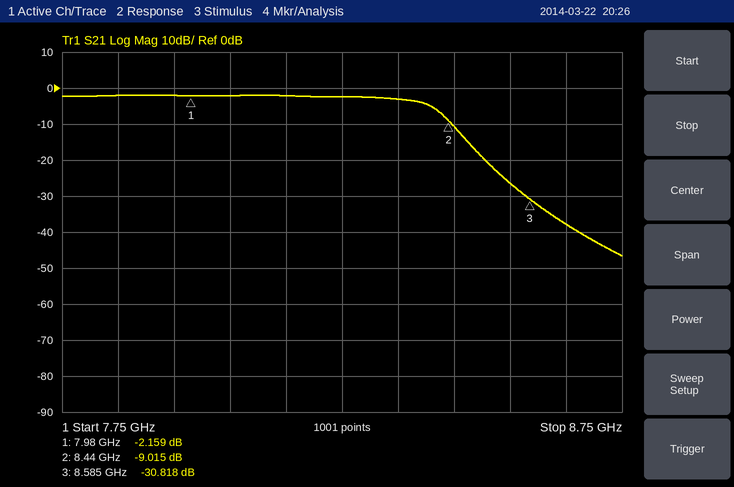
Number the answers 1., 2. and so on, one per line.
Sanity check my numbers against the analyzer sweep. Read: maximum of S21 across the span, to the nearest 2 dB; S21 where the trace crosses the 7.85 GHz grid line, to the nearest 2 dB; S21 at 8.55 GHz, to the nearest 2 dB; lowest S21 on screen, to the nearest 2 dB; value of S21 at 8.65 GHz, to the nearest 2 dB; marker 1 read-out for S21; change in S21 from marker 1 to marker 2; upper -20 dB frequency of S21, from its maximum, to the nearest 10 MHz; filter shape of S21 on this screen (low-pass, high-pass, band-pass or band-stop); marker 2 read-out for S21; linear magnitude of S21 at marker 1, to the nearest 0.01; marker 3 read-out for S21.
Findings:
1. -2 dB
2. -2 dB
3. -26 dB
4. -46 dB
5. -38 dB
6. -2.159 dB
7. -6.856 dB
8. 8.52 GHz
9. low-pass
10. -9.015 dB
11. 0.78
12. -30.818 dB
